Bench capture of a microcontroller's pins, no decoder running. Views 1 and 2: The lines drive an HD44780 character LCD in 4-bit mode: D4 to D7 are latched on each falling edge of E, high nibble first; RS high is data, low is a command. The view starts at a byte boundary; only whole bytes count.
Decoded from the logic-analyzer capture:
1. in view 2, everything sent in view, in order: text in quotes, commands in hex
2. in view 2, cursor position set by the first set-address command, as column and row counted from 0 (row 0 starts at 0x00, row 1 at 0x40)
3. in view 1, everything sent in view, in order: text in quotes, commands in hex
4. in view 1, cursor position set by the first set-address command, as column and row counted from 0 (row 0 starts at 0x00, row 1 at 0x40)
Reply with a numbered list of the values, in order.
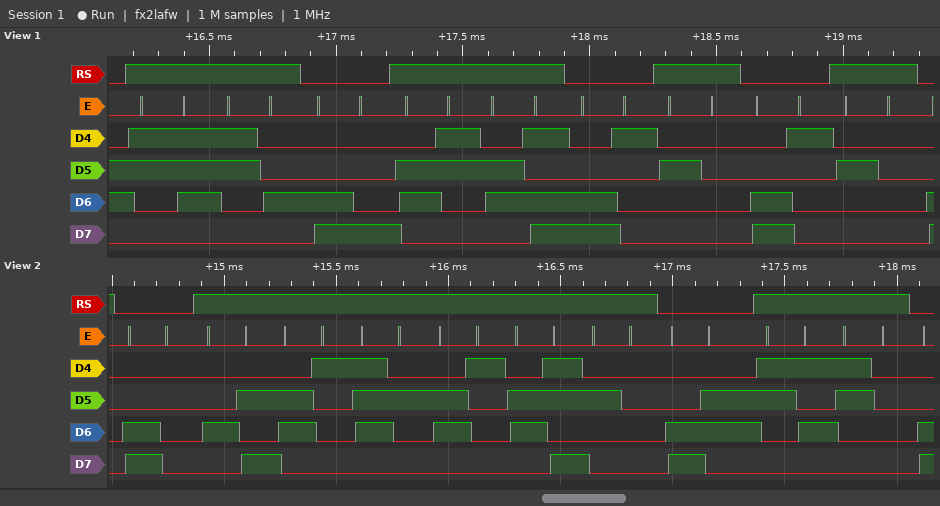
1. 0xC0 "Jarak " 0xC6 "50"
2. column 0, row 1
3. "74" 0xC8 "cm" 0xC1 " " 0xC1 " "
4. column 8, row 1
